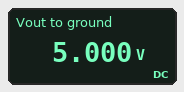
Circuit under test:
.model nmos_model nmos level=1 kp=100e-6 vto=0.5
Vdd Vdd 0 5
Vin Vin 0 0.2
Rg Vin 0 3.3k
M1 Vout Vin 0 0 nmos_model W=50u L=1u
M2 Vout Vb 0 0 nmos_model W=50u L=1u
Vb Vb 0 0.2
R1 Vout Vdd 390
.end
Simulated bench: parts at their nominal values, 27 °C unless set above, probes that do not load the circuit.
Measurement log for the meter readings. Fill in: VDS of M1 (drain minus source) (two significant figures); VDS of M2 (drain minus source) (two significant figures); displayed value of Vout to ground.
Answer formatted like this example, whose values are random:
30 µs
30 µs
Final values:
5.0 V
5.0 V
5.000 V
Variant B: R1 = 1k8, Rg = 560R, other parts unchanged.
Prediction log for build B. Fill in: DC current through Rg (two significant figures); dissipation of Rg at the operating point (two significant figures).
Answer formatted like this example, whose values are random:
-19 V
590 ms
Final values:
360 µA
71 µW
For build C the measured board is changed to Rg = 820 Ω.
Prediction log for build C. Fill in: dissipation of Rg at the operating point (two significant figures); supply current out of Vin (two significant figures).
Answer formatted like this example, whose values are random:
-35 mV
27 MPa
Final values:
49 µW
240 µA
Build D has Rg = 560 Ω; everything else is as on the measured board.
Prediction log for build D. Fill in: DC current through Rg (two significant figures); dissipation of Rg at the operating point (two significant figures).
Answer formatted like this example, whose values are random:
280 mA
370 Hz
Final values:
360 µA
71 µW
